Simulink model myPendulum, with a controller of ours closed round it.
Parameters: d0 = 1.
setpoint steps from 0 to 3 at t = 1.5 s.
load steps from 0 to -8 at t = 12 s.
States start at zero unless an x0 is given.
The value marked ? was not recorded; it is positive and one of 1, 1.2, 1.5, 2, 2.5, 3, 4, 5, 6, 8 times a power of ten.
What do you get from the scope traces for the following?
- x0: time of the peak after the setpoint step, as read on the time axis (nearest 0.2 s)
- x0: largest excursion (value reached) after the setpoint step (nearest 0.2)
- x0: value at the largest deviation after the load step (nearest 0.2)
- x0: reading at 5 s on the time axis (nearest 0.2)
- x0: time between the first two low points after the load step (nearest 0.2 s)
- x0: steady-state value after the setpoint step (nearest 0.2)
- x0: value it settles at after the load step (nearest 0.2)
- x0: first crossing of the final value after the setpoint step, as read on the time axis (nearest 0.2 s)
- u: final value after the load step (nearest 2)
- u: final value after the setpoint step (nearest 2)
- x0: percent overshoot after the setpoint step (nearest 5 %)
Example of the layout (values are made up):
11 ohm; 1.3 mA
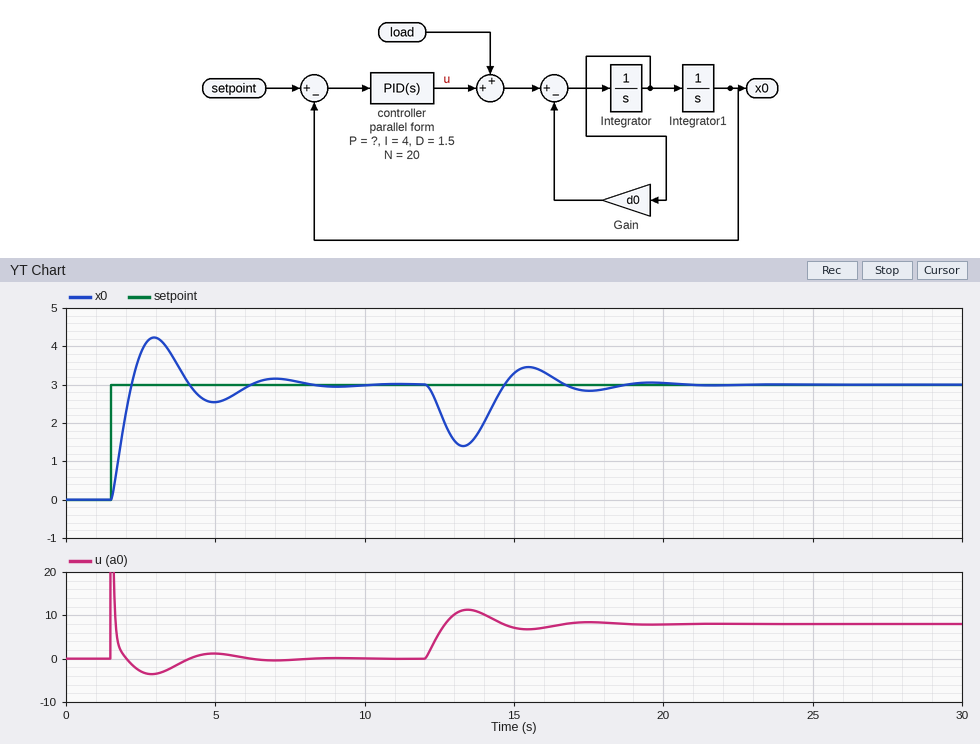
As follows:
3.0 s; 4.2; 1.4; 2.6; 4.2 s; 3.0; 3.0; 2.2 s; 8; 0; 40 %
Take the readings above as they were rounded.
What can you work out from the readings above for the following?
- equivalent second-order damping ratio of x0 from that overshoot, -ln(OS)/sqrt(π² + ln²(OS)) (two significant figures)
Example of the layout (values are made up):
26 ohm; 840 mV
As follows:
0.28
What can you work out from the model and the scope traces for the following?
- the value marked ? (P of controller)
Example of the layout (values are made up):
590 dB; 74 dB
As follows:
4
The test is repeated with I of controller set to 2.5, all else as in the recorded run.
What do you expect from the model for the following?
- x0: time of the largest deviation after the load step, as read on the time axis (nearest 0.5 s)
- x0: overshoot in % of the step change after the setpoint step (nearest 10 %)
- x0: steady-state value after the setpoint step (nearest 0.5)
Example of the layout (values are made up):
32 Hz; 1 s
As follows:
13.5 s; 30 %; 3.0
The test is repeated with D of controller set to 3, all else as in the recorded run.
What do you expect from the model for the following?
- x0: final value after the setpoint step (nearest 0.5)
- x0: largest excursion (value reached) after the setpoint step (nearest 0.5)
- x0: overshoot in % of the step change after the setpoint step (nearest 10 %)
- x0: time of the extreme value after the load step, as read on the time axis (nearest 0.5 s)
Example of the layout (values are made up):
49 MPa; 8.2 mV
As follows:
3.0; 3.5; 20 %; 13.5 s
